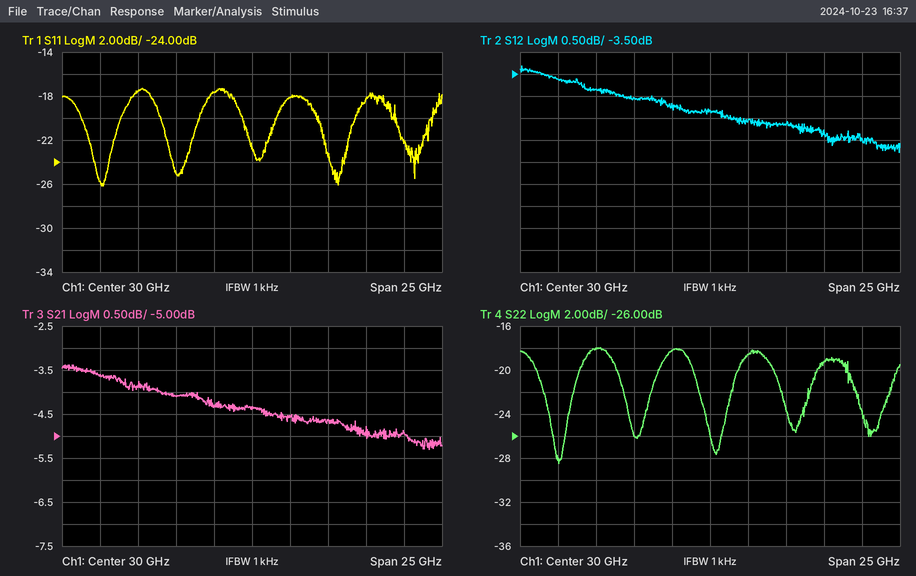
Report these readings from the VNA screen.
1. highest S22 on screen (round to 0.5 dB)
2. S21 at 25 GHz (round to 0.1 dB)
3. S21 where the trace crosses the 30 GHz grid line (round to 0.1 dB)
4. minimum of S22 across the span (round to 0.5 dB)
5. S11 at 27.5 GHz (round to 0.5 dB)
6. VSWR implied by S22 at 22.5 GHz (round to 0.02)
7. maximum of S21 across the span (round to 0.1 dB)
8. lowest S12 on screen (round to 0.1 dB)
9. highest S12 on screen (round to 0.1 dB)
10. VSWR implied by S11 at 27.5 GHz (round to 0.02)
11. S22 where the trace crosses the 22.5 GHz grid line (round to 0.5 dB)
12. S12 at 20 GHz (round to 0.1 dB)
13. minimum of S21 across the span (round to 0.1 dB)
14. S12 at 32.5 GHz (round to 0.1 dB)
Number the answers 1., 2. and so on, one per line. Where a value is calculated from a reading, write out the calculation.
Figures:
1. -18.0 dB
2. -4.1 dB
3. -4.4 dB
4. -28.5 dB
5. -17.5 dB
6. |Γ| = 10^(-18/20) = 0.1259; VSWR = (1 + 0.1259)/(1 − 0.1259) ≈ 1.29, so 1.28 to the nearest 0.02
7. -3.4 dB
8. -5.3 dB
9. -3.3 dB
10. |Γ| = 10^(-17.5/20) = 0.1334; VSWR = (1 + 0.1334)/(1 − 0.1334) ≈ 1.31, so 1.30 to the nearest 0.02
11. -18.0 dB
12. -3.6 dB
13. -5.3 dB
14. -4.6 dB
